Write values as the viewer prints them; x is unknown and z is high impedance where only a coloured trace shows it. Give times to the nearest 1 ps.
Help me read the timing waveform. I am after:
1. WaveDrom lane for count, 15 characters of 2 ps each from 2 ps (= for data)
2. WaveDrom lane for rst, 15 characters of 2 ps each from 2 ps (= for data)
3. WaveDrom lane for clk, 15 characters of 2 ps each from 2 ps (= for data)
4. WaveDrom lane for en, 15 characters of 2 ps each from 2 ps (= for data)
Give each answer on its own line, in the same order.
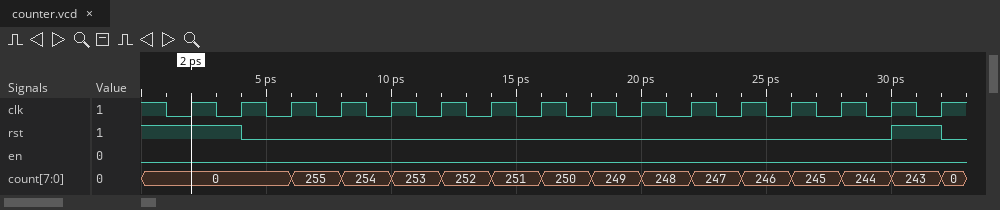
{name: 'count', wave: '=.=============', data: '0 255 254 253 252 251 250 249 248 247 246 245 244 243'}
{name: 'rst', wave: '10............1'}
{name: 'clk', wave: 'p..............'}
{name: 'en', wave: '0..............'}
